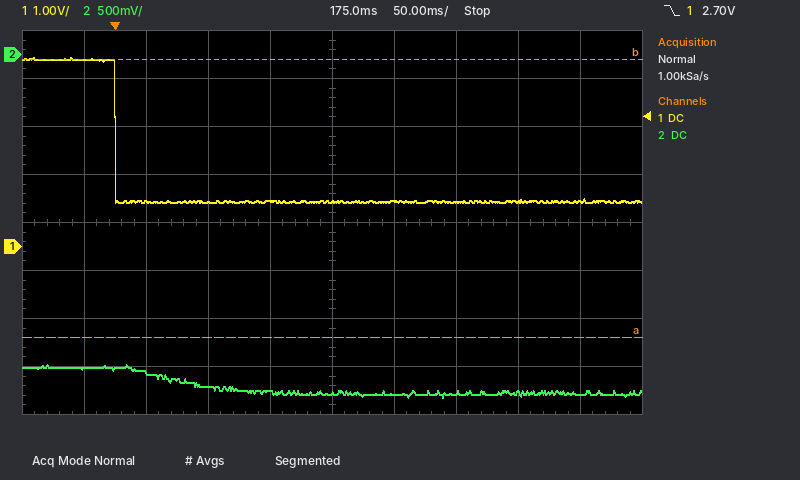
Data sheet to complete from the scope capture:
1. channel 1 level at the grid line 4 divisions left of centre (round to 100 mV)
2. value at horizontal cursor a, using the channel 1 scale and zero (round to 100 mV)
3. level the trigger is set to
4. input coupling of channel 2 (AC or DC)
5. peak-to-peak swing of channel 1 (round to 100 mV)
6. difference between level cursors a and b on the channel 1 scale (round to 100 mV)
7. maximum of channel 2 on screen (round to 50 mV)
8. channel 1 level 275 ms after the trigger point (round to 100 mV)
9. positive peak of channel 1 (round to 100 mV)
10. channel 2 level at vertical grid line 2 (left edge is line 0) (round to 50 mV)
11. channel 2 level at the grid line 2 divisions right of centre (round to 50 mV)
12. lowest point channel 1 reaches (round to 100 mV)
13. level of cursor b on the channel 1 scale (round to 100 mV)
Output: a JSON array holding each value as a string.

["3.9 V", "-1.9 V", "2.70 V", "DC", "3.0 V", "5.8 V", "-3.25 V", "900 mV", "3.9 V", "-3.30 V", "-3.50 V", "900 mV", "3.9 V"]
